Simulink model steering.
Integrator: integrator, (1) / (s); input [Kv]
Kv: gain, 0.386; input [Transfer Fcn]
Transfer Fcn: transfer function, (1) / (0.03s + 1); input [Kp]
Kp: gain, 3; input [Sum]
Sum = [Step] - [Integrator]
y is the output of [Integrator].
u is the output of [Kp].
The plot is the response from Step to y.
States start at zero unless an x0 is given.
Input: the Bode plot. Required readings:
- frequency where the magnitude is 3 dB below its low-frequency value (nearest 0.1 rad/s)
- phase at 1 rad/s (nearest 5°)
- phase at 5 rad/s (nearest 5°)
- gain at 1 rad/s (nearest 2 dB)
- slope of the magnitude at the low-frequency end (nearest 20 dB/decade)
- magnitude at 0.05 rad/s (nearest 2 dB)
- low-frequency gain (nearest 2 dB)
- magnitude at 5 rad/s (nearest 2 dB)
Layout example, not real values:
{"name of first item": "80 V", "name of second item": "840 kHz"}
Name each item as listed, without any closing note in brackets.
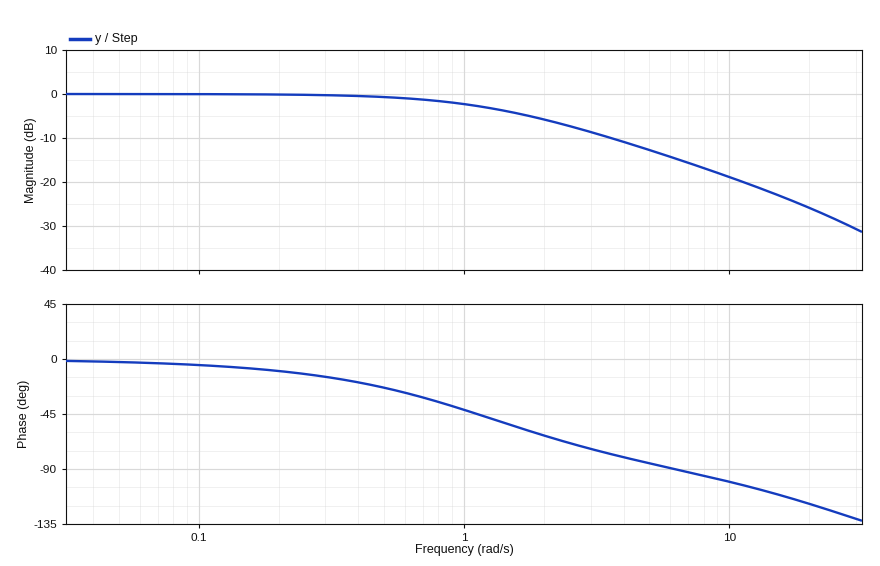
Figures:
{"frequency where the magnitude is 3 dB below its low-frequency value": "1.2 rad/s", "phase at 1 rad/s": "-40°", "phase at 5 rad/s": "-85°", "gain at 1 rad/s": "-2 dB", "slope of the magnitude at the low-frequency end": "0 dB/decade", "magnitude at 0.05 rad/s": "0 dB", "low-frequency gain": "0 dB", "magnitude at 5 rad/s": "-12 dB"}
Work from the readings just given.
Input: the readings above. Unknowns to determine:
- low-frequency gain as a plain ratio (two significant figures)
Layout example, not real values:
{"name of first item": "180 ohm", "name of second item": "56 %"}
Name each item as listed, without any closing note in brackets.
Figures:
{"low-frequency gain as a plain ratio": "1.0"}
